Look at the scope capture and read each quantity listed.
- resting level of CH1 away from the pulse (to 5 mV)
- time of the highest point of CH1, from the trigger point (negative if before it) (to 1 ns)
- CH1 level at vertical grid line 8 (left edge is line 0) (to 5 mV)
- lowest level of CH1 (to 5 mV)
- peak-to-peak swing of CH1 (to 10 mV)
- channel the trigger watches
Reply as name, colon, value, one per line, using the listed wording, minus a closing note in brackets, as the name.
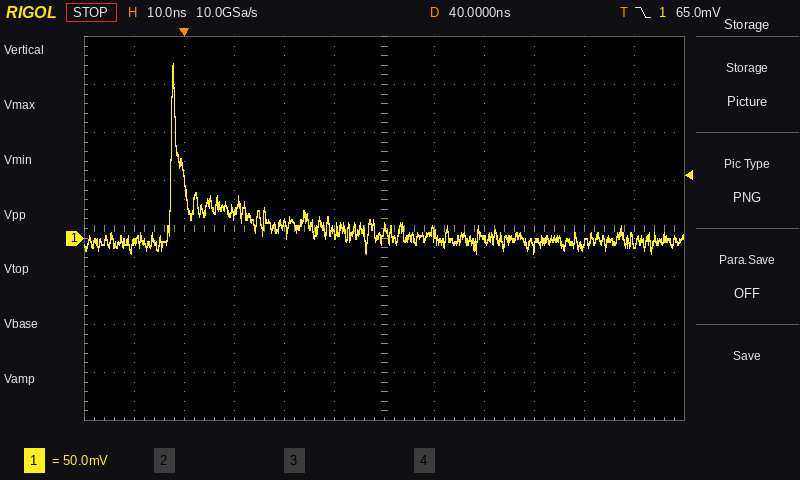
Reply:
resting level of CH1 away from the pulse: 0 mV
time of the highest point of CH1, from the trigger point (negative if before it): -2 ns
CH1 level at vertical grid line 8 (left edge is line 0): 0 mV
lowest level of CH1: -15 mV
peak-to-peak swing of CH1: 200 mV
channel the trigger watches: CH1
